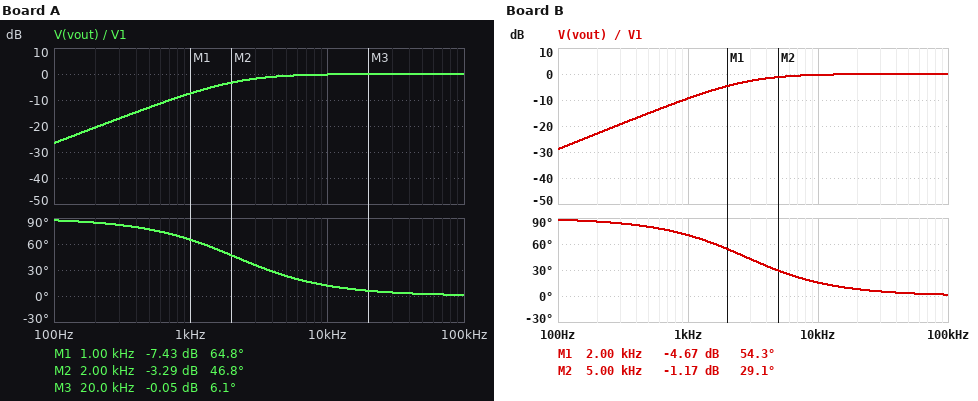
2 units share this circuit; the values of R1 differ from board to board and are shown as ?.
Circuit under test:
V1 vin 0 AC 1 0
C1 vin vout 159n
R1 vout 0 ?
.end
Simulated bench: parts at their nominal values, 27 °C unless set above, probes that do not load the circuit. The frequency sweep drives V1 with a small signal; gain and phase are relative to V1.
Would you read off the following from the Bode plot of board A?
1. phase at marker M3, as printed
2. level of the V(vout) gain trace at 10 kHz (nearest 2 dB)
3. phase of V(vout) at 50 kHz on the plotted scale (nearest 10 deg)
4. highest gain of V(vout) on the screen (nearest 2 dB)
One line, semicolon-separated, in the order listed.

6.1 deg; 0 dB; 0 deg; 0 dB
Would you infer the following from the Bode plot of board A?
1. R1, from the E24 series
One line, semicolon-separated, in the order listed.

470 Ω
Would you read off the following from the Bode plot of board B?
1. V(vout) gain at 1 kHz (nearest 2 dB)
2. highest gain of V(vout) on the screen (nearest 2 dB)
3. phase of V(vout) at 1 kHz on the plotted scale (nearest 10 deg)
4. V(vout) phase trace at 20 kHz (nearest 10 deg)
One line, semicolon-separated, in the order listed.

-10 dB; 0 dB; 70 deg; 10 deg
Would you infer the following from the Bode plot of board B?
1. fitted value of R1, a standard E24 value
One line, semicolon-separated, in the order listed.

360 Ω
